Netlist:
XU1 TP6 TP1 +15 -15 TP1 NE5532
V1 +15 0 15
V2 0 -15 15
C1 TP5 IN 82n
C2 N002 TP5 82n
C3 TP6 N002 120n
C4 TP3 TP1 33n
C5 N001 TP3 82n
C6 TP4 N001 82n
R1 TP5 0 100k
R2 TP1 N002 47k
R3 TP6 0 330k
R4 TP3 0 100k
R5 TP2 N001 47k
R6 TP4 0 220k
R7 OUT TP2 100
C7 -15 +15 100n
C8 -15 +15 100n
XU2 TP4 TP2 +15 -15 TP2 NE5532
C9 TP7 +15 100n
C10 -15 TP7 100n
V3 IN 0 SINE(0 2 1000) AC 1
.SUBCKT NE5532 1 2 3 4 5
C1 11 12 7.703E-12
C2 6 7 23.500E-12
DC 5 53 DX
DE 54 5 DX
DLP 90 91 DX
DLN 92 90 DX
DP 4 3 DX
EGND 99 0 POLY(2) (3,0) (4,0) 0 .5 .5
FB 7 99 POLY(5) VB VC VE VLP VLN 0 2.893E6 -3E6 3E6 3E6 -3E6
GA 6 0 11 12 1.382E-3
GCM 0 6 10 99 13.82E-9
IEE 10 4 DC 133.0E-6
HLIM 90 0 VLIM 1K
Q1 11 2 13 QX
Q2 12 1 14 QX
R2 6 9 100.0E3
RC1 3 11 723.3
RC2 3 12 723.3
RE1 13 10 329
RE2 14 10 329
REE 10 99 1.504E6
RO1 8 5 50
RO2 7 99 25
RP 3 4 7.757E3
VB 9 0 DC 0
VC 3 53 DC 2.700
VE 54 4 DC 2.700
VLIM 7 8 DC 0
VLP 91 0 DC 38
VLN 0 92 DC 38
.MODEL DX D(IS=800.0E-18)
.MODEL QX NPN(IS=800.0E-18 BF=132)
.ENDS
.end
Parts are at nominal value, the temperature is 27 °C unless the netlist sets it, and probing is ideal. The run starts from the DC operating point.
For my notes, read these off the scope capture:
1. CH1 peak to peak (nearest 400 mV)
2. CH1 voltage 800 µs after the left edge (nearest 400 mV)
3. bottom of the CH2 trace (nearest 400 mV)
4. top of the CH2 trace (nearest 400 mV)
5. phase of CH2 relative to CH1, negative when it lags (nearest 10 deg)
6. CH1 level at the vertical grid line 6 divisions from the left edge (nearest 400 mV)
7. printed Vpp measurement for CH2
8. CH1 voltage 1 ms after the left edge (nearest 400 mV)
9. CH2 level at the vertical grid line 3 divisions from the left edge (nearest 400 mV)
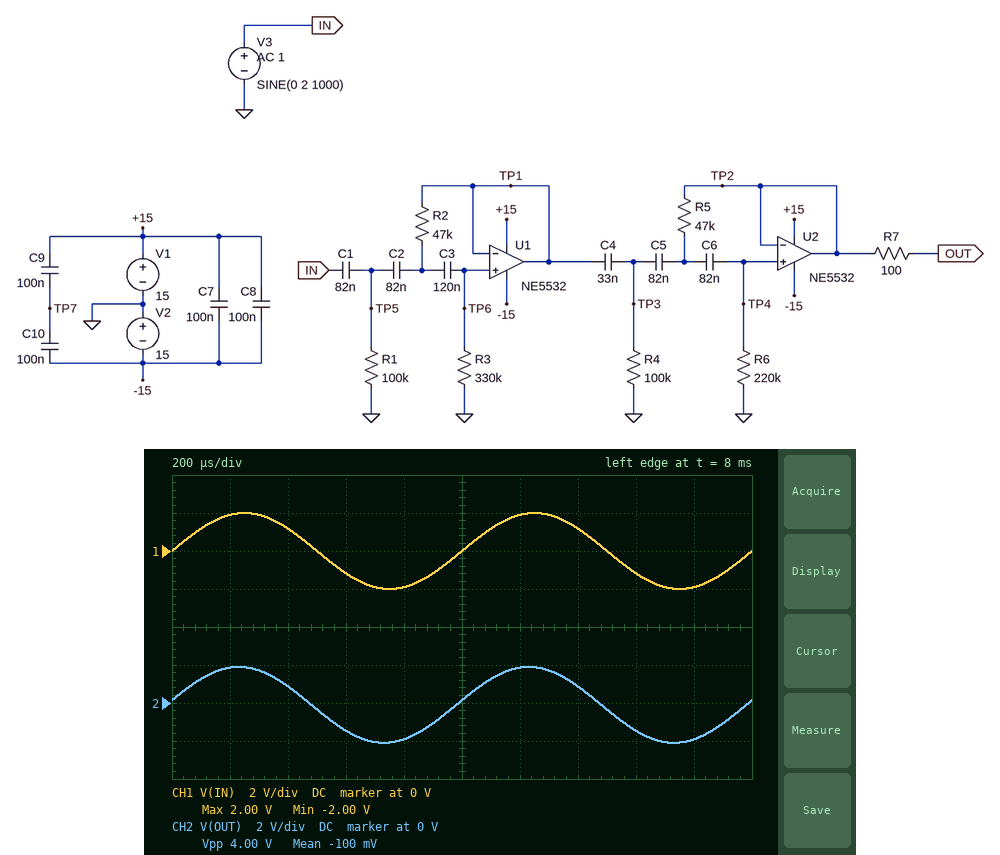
4.0 V
-2.0 V
-2.0 V
2.0 V
10 deg
2.0 V
4.00 V
0 V
-1.6 V
